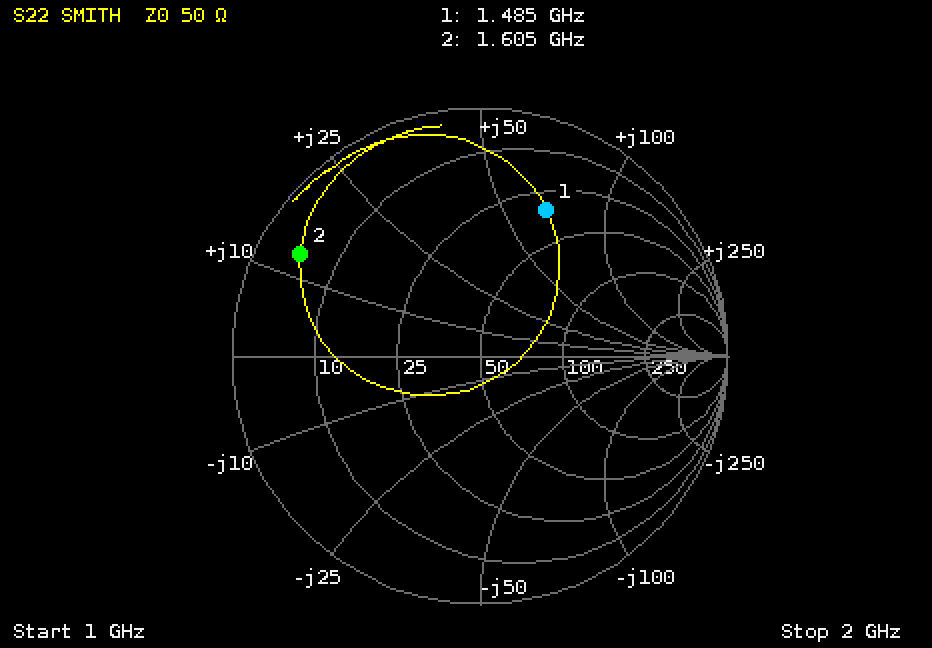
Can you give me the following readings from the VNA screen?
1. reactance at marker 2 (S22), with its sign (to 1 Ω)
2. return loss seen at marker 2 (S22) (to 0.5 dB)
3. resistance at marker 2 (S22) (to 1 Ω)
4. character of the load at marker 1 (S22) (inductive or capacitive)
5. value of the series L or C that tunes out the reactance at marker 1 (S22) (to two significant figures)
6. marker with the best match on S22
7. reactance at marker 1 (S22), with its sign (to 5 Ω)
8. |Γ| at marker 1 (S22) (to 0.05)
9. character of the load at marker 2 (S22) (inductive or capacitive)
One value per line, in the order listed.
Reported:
+13 Ω
1.5 dB
5 Ω
inductive
1.6 pF
marker 1
+65 Ω
0.65
inductive
